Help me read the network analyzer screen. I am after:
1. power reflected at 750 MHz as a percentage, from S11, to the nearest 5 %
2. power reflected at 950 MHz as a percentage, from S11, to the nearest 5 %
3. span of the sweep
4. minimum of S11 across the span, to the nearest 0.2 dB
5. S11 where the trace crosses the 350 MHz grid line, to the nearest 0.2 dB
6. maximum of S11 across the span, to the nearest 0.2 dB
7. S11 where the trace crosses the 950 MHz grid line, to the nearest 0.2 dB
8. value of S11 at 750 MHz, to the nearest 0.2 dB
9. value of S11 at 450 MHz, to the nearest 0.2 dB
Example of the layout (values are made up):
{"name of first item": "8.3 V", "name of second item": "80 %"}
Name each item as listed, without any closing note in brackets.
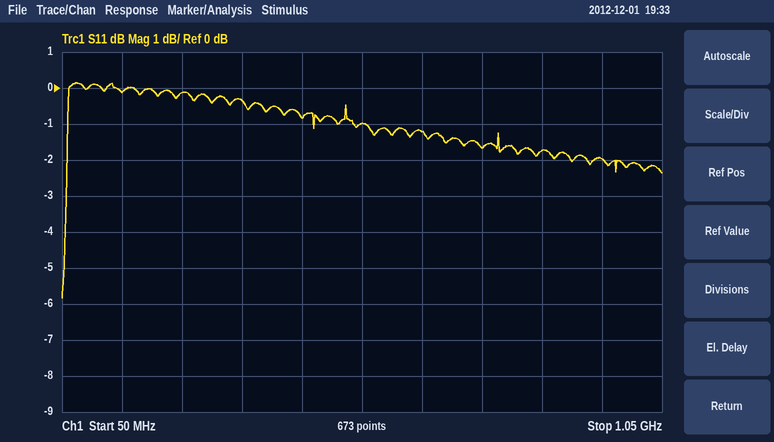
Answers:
{"power reflected at 750 MHz as a percentage, from S11, to the nearest 5 %": "70 %", "power reflected at 950 MHz as a percentage, from S11, to the nearest 5 %": "65 %", "span of the sweep": "1 GHz", "minimum of S11 across the span, to the nearest 0.2 dB": "-5.8 dB", "S11 where the trace crosses the 350 MHz grid line, to the nearest 0.2 dB": "-0.4 dB", "maximum of S11 across the span, to the nearest 0.2 dB": "0.2 dB", "S11 where the trace crosses the 950 MHz grid line, to the nearest 0.2 dB": "-2.0 dB", "value of S11 at 750 MHz, to the nearest 0.2 dB": "-1.6 dB", "value of S11 at 450 MHz, to the nearest 0.2 dB": "-0.8 dB"}
